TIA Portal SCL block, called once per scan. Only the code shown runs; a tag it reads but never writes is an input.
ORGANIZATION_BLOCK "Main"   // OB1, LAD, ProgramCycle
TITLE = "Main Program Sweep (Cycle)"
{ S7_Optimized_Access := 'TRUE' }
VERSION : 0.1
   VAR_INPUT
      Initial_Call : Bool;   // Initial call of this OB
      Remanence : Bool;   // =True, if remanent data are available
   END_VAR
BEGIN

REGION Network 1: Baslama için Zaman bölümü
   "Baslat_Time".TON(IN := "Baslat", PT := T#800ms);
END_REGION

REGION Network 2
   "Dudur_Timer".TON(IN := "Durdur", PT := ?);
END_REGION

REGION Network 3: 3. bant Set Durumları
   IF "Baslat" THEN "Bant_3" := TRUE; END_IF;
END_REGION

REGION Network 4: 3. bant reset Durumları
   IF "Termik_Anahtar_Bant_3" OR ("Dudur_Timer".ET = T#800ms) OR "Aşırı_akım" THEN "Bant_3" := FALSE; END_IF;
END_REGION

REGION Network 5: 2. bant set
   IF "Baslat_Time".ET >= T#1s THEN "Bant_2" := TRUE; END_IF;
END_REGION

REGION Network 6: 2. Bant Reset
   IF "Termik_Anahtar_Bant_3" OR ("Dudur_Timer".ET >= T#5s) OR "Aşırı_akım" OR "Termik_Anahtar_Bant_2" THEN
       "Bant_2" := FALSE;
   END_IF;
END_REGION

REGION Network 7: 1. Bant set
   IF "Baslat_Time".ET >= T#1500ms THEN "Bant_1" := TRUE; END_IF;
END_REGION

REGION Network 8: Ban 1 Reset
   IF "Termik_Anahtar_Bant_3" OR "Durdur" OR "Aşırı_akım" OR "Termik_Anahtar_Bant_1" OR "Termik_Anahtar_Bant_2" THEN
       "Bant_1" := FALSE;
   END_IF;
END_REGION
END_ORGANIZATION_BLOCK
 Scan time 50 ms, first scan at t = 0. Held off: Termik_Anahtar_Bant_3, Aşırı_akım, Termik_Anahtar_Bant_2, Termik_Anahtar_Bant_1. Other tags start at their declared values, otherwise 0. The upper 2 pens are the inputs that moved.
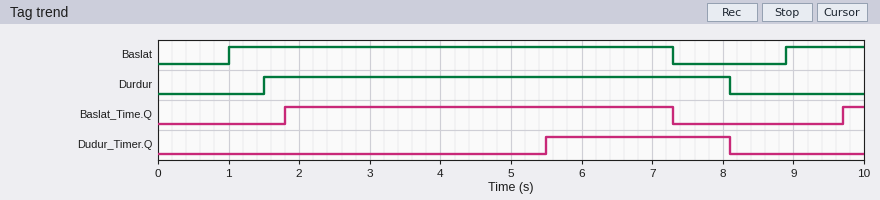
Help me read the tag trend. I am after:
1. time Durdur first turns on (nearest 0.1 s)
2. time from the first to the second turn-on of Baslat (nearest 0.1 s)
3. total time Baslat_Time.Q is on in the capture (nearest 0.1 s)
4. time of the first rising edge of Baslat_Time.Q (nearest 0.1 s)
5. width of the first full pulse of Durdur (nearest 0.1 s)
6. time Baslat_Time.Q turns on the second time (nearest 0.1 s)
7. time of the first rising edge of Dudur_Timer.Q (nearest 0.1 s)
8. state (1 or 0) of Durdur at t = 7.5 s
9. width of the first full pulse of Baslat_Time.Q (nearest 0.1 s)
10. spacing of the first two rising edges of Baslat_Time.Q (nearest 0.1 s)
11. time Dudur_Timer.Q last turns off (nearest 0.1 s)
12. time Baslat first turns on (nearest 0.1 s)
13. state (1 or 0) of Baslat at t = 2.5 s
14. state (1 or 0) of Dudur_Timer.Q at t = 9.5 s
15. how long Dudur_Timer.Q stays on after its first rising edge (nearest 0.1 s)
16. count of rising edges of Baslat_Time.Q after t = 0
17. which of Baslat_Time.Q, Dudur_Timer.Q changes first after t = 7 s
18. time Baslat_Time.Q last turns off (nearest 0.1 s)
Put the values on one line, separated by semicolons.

1.5 s; 7.9 s; 5.8 s; 1.8 s; 6.6 s; 9.7 s; 5.5 s; 1; 5.5 s; 7.9 s; 8.1 s; 1.0 s; 1; 0; 2.6 s; 2; Baslat_Time.Q; 7.3 s
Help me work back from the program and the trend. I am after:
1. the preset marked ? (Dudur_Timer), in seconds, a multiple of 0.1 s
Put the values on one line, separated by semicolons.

4.0 s
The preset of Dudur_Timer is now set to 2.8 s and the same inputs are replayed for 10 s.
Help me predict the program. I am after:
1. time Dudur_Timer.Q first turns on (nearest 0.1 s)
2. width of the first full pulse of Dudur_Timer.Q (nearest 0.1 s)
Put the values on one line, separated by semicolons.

4.3 s; 3.8 s
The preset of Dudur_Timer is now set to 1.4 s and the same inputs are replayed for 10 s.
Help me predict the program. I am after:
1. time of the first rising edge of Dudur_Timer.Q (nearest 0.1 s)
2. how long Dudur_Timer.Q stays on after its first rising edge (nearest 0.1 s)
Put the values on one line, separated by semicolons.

2.9 s; 5.2 s
